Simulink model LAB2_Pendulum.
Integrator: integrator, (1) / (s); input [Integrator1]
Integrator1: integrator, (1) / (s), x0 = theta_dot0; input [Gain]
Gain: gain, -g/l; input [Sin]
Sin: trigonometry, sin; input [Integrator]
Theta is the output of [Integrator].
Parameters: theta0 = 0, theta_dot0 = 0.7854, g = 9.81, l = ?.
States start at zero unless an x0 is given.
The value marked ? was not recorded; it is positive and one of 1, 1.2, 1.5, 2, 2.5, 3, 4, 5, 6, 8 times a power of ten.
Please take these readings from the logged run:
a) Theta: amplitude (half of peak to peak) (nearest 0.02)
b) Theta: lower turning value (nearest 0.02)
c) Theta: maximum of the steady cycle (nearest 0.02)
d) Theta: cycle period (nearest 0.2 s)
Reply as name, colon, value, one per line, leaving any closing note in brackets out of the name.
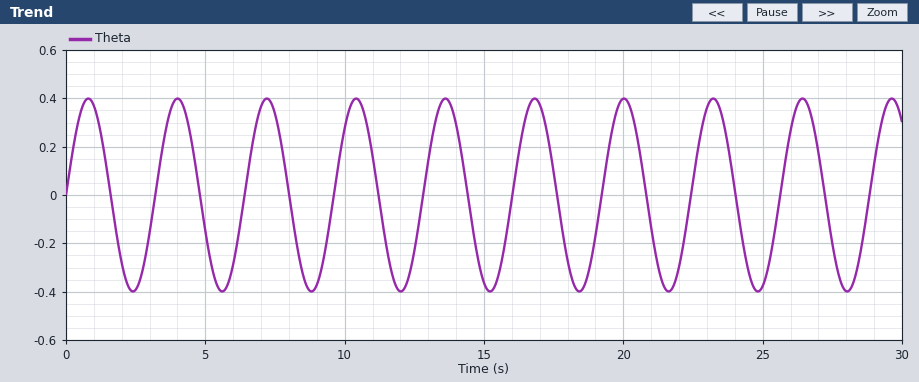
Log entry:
Theta: amplitude (half of peak to peak): 0.40
Theta: lower turning value: -0.40
Theta: maximum of the steady cycle: 0.40
Theta: cycle period: 3.2 s
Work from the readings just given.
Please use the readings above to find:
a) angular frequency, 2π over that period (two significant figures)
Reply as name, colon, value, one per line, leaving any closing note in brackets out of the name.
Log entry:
angular frequency, 2π over that period: 2.0 rad/s
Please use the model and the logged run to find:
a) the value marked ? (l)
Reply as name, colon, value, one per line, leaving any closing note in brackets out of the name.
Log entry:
the value marked ?: 2.5
